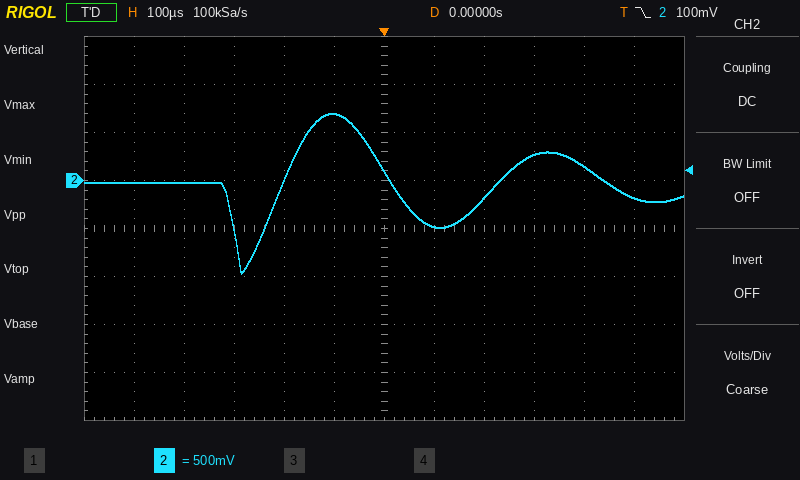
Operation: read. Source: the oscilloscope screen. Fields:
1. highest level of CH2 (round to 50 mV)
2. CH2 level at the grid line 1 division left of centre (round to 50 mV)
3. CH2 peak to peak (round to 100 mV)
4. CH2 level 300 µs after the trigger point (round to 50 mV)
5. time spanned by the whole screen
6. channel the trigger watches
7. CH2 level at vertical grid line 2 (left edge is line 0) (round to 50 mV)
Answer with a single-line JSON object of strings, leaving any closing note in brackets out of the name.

{"highest level of CH2": "700 mV", "CH2 level at the grid line 1 division left of centre": "700 mV", "CH2 peak to peak": "1.70 V", "CH2 level 300 µs after the trigger point": "250 mV", "time spanned by the whole screen": "1.2 ms", "channel the trigger watches": "CH2", "CH2 level at vertical grid line 2 (left edge is line 0)": "0 mV"}
